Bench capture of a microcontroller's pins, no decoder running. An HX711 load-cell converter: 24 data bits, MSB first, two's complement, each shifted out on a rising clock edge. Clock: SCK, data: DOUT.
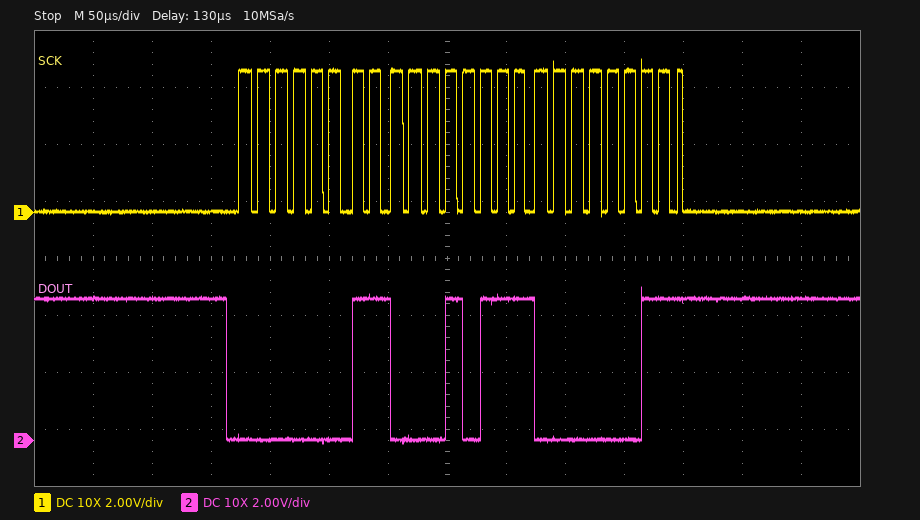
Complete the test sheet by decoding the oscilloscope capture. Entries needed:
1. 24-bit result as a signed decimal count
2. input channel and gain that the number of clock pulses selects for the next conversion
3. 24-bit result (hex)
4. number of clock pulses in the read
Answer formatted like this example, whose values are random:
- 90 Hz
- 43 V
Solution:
- 202499
- channel A, gain 128
- 0x031703
- 25
